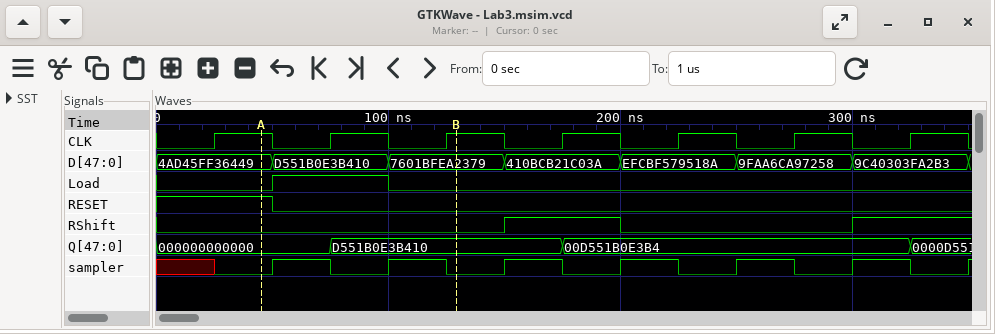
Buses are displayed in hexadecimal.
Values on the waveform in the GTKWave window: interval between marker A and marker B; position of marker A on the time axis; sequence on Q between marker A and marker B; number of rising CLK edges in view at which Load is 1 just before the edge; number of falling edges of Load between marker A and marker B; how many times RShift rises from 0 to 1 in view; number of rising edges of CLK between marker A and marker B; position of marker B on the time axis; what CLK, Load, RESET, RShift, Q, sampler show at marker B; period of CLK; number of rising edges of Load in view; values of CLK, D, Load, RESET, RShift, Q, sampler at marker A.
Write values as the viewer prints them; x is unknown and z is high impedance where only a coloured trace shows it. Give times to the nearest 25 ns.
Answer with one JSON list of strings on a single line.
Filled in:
["75 ns", "50 ns", "000000000000, D551B0E3B410", "1", "1", "2", "2", "125 ns", "CLK=1, Load=0, RESET=0, RShift=0, Q=D551B0E3B410, sampler=0", "50 ns", "1", "CLK=1, D=4AD45FF36449, Load=0, RESET=1, RShift=0, Q=000000000000, sampler=0"]
